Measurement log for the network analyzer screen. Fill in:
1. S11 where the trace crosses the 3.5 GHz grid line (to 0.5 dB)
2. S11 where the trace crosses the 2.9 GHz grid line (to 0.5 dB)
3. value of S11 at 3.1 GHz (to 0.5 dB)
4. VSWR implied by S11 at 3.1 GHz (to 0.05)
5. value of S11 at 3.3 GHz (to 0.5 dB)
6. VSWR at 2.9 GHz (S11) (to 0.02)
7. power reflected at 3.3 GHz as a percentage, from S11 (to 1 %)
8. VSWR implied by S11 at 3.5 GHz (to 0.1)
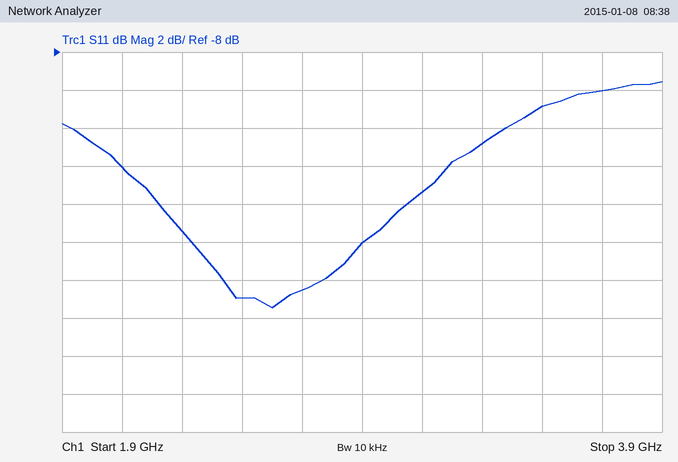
-11.0 dB
-18.0 dB
-15.5 dB
1.40
-13.0 dB
1.28
5 %
1.8
